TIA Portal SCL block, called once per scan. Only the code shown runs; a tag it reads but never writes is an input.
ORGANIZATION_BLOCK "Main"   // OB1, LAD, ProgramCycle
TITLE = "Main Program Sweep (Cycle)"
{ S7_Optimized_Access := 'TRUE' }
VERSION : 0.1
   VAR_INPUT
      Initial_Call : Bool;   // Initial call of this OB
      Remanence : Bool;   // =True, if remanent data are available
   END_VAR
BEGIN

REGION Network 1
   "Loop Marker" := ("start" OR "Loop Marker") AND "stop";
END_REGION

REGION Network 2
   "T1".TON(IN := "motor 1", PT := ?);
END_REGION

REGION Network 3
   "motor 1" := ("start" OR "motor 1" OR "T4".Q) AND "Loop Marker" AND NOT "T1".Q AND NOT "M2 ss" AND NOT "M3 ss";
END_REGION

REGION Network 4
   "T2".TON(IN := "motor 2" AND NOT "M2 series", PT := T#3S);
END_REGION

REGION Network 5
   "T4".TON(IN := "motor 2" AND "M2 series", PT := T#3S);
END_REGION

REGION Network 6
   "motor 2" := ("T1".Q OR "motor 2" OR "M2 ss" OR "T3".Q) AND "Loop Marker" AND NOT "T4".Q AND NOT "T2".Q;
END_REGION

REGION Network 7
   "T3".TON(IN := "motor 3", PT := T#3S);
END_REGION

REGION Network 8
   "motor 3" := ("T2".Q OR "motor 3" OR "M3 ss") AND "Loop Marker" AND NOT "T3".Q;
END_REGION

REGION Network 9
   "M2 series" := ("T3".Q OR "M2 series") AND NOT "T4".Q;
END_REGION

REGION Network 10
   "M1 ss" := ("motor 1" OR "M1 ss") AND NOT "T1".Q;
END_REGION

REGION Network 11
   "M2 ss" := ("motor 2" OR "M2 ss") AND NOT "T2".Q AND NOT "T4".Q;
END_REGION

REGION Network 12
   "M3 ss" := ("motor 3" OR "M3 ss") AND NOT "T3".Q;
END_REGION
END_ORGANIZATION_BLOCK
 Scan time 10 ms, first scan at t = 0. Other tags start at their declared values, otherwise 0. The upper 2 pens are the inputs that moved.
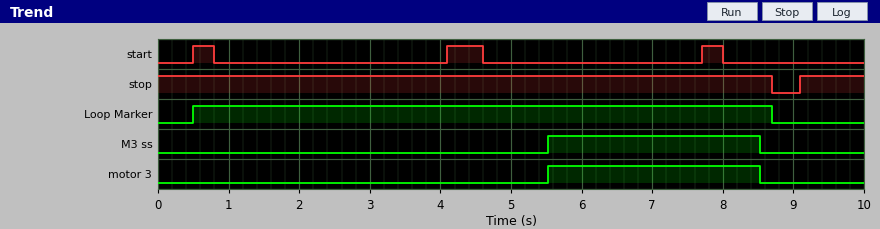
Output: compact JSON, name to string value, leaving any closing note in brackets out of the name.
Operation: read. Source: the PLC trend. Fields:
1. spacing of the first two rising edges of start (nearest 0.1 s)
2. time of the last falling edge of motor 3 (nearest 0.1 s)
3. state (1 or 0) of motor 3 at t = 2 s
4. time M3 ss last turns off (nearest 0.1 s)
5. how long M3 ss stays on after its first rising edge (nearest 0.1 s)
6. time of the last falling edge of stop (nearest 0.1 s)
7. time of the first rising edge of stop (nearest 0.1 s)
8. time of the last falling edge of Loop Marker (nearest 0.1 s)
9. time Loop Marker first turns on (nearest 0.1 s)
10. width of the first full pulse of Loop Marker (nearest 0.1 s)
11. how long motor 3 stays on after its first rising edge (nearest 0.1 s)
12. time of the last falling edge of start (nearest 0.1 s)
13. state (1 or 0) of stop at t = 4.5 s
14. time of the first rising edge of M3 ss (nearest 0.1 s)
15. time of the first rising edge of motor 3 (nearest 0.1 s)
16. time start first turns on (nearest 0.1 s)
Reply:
{"spacing of the first two rising edges of start": "3.6 s", "time of the last falling edge of motor 3": "8.5 s", "state (1 or 0) of motor 3 at t = 2 s": "0", "time M3 ss last turns off": "8.5 s", "how long M3 ss stays on after its first rising edge": "3.0 s", "time of the last falling edge of stop": "8.7 s", "time of the first rising edge of stop": "9.1 s", "time of the last falling edge of Loop Marker": "8.7 s", "time Loop Marker first turns on": "0.5 s", "width of the first full pulse of Loop Marker": "8.2 s", "how long motor 3 stays on after its first rising edge": "3.0 s", "time of the last falling edge of start": "8.0 s", "state (1 or 0) of stop at t = 4.5 s": "1", "time of the first rising edge of M3 ss": "5.5 s", "time of the first rising edge of motor 3": "5.5 s", "time start first turns on": "0.5 s"}
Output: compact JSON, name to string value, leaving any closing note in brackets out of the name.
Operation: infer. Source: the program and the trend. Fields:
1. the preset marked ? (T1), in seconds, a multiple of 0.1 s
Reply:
{"the preset marked ? (T1), in seconds, a multiple of 0.1 s": "2.0 s"}
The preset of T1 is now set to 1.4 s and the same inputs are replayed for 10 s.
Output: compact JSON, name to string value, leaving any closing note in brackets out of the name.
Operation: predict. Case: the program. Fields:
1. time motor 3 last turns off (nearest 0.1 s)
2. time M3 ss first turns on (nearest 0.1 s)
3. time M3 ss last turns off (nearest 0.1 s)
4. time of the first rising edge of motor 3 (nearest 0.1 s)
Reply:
{"time motor 3 last turns off": "7.9 s", "time M3 ss first turns on": "4.9 s", "time M3 ss last turns off": "7.9 s", "time of the first rising edge of motor 3": "4.9 s"}
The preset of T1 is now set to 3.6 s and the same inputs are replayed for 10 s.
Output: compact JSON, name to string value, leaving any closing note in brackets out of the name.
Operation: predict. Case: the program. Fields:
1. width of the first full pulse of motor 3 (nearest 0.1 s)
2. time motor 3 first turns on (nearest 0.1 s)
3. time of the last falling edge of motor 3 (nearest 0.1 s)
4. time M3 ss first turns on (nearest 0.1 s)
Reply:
{"width of the first full pulse of motor 3": "1.6 s", "time motor 3 first turns on": "7.1 s", "time of the last falling edge of motor 3": "8.7 s", "time M3 ss first turns on": "7.1 s"}
